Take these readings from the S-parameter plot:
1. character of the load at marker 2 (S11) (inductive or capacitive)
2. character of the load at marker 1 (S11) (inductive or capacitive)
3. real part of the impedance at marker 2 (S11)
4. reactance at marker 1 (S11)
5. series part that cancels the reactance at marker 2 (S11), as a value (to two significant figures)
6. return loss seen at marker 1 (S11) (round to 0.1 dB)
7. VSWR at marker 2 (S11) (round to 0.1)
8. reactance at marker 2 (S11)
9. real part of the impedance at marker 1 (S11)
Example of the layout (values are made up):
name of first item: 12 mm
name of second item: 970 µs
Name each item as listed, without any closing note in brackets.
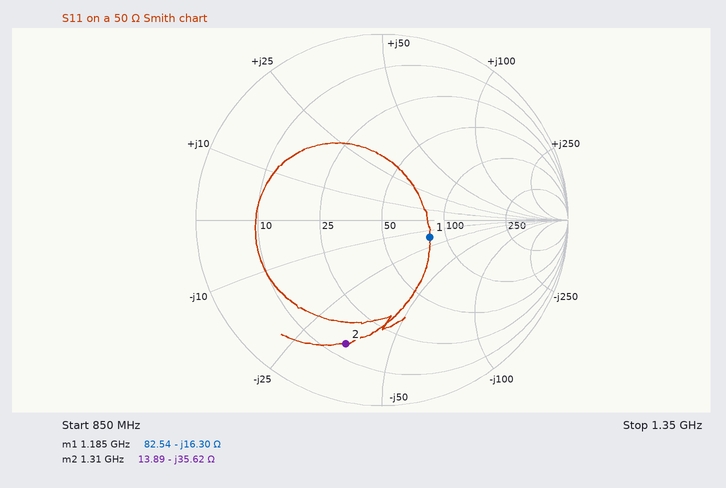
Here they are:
character of the load at marker 2 (S11): capacitive
character of the load at marker 1 (S11): capacitive
real part of the impedance at marker 2: 13.89 Ω
reactance at marker 1: -16.30 Ω
series part that cancels the reactance at marker 2 (S11), as a value: 4.3 nH
return loss seen at marker 1 (S11): 11.3 dB
VSWR at marker 2 (S11): 5.5
reactance at marker 2: -35.62 Ω
real part of the impedance at marker 1: 82.54 Ω
